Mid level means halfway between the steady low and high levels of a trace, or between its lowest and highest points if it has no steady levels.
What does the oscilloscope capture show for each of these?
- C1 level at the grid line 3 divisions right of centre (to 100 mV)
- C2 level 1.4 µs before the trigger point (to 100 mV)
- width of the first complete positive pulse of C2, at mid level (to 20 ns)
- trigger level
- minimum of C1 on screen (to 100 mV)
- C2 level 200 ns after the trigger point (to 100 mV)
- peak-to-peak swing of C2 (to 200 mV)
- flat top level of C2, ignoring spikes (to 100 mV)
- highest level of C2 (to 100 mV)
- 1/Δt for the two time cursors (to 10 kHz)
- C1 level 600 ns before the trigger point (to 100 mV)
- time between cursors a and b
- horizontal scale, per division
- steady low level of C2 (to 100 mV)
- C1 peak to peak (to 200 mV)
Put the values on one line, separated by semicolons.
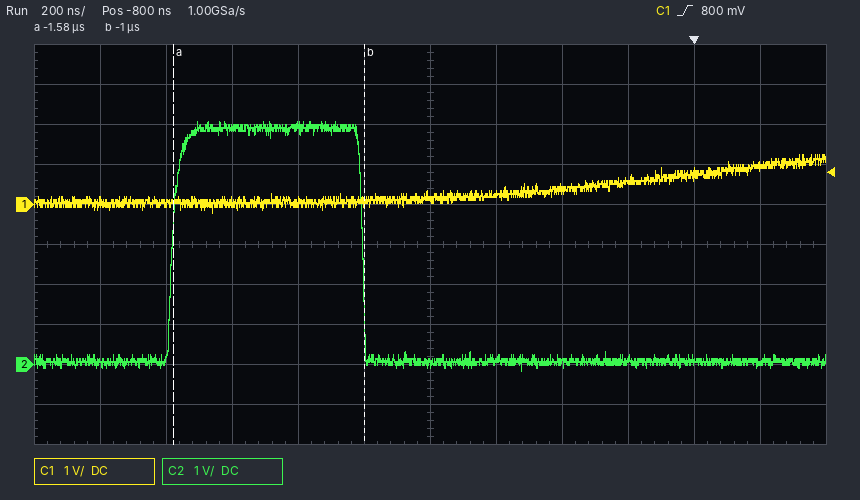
600 mV; 5.9 V; 580 ns; 800 mV; -200 mV; 100 mV; 6.2 V; 5.9 V; 6.1 V; 1.72 MHz; 300 mV; 580 ns; 200 ns; 100 mV; 1.4 V
